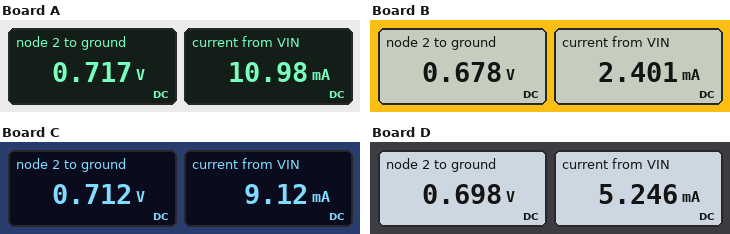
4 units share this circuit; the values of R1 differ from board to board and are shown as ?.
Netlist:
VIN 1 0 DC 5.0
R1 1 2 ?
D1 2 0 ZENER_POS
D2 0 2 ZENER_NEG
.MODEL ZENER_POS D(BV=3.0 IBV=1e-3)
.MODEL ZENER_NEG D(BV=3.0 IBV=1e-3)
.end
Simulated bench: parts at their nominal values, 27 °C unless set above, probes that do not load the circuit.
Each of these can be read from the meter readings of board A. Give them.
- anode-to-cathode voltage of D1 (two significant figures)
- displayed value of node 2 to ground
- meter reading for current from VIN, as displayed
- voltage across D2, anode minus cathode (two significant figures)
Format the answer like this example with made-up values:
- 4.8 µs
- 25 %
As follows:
- 720 mV
- 0.717 V
- 10.98 mA
- -720 mV
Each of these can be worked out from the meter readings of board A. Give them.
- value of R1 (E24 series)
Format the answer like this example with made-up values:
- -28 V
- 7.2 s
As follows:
- 390 Ω
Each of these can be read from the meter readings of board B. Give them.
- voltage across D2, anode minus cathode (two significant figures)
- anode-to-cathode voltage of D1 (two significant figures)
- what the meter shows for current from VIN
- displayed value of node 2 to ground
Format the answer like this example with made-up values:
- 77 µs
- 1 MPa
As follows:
- -680 mV
- 680 mV
- 2.401 mA
- 0.678 V
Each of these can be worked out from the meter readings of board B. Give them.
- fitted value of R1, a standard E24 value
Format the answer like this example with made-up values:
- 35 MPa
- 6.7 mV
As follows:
- 1.8 kΩ
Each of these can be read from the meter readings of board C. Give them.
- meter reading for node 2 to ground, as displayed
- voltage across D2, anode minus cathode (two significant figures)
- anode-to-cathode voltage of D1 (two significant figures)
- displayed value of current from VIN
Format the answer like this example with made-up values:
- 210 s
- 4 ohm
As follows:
- 0.712 V
- -710 mV
- 710 mV
- 9.12 mA
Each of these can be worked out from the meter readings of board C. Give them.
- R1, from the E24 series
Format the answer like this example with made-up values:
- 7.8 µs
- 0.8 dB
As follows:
- 470 Ω
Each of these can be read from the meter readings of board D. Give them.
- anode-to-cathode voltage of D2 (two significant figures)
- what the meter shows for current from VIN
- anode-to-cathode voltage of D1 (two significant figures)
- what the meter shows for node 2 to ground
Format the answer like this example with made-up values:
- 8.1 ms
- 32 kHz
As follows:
- -700 mV
- 5.246 mA
- 700 mV
- 0.698 V
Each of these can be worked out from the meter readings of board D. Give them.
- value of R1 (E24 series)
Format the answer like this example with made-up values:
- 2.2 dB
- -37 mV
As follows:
- 820 Ω
